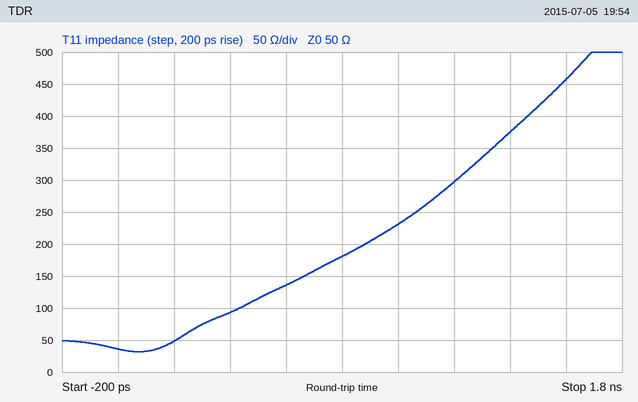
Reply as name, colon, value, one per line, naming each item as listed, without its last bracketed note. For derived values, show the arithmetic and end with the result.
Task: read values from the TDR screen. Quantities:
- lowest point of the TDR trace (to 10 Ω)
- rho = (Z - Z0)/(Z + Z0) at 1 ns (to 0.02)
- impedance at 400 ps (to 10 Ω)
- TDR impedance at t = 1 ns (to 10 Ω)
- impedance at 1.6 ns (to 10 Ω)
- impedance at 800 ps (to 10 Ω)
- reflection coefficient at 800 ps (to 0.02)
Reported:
lowest point of the TDR trace: 30 Ω
rho = (Z - Z0)/(Z + Z0) at 1 ns: (230 − 50)/(230 + 50) ≈ +0.64
impedance at 400 ps: 90 Ω
TDR impedance at t = 1 ns: 230 Ω
impedance at 1.6 ns: 460 Ω
impedance at 800 ps: 180 Ω
reflection coefficient at 800 ps: (180 − 50)/(180 + 50) ≈ +0.56
